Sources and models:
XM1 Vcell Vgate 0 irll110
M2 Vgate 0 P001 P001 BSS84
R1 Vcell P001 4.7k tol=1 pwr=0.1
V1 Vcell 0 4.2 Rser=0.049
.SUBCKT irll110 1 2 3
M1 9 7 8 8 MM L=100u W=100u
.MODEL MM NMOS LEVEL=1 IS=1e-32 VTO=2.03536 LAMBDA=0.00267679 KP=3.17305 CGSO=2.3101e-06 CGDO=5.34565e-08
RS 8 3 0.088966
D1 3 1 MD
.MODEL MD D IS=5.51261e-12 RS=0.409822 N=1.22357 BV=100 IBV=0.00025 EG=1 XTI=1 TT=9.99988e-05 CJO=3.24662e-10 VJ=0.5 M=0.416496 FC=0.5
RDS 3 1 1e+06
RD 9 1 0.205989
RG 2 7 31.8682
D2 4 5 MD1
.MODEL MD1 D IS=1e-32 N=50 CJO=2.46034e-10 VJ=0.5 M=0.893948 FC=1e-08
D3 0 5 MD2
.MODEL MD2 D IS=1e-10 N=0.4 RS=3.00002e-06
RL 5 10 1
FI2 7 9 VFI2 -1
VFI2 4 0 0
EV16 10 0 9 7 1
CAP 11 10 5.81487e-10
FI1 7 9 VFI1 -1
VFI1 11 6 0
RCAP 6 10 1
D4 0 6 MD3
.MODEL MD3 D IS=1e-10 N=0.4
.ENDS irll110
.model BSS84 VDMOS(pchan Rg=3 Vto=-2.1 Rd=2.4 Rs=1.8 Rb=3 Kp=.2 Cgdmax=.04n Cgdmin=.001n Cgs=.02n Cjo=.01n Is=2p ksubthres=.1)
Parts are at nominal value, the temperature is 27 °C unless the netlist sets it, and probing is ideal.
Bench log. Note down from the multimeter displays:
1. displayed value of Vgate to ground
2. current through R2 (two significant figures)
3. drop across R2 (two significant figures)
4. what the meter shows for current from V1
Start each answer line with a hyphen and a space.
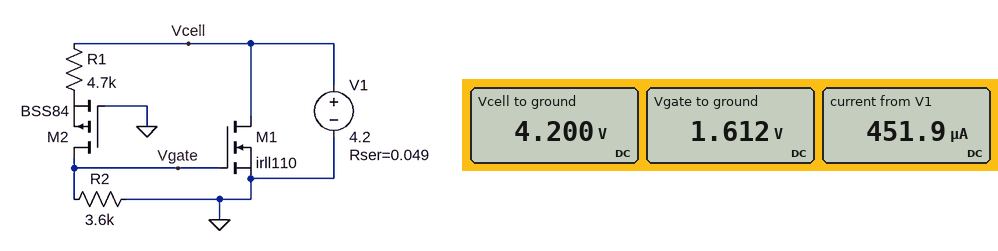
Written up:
- 1.612 V
- 450 µA
- 1.6 V
- 451.9 µA
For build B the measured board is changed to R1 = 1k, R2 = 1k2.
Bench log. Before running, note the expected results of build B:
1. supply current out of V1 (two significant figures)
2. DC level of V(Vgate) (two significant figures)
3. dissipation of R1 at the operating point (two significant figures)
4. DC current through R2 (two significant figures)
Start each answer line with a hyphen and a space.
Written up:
- 77 mA
- 2.3 V
- 3.5 mW
- 1.9 mA
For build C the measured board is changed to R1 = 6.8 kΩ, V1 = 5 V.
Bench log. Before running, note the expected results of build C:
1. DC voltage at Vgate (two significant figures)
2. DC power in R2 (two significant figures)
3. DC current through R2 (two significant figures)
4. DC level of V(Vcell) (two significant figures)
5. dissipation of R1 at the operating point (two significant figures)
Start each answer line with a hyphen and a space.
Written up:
- 1.5 V
- 660 µW
- 430 µA
- 5.0 V
- 1.2 mW
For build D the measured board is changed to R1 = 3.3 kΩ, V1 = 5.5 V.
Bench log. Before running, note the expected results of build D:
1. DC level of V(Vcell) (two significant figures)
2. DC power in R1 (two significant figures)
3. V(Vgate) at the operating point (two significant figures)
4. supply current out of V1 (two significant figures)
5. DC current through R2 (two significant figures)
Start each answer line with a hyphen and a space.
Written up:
- 5.5 V
- 2.1 mW
- 2.8 V
- 860 mA
- 790 µA
